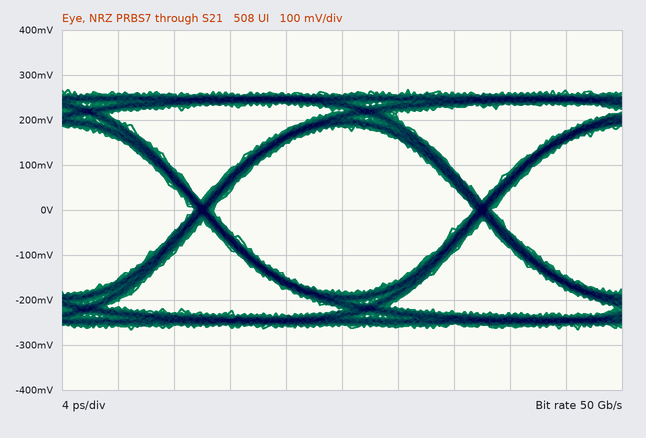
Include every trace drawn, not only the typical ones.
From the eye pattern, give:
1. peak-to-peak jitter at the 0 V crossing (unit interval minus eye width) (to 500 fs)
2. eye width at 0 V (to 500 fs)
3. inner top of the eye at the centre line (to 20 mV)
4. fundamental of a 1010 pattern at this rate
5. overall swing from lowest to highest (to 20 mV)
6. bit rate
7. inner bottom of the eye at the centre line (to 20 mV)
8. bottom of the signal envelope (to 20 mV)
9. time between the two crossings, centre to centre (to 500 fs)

1.5 ps
18.5 ps
180 mV
25 GHz
540 mV
50 Gb/s
-180 mV
-260 mV
20.0 ps
